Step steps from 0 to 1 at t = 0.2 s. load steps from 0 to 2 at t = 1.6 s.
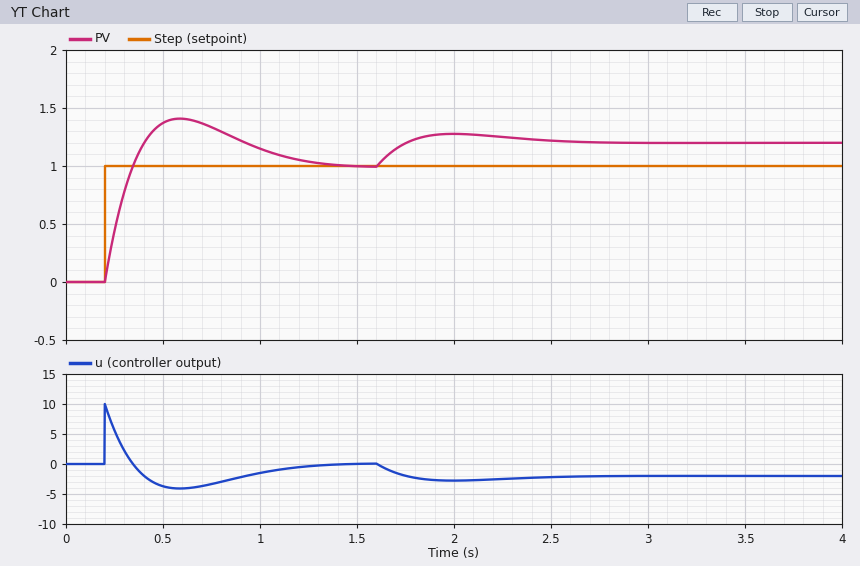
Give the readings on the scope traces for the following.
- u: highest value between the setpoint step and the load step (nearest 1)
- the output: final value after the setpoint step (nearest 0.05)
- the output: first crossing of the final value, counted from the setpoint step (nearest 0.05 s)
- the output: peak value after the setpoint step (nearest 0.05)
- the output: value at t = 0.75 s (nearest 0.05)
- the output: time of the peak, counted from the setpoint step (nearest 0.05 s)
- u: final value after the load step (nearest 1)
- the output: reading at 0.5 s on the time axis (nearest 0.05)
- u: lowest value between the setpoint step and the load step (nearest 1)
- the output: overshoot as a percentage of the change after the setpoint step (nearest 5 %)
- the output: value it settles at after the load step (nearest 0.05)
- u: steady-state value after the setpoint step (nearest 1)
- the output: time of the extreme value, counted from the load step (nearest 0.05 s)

10
1.00
0.15 s
1.40
1.35
0.40 s
-2
1.35
-4
40 %
1.20
0
0.40 s
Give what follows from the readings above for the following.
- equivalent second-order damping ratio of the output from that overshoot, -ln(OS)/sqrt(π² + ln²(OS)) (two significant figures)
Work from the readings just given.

0.28
